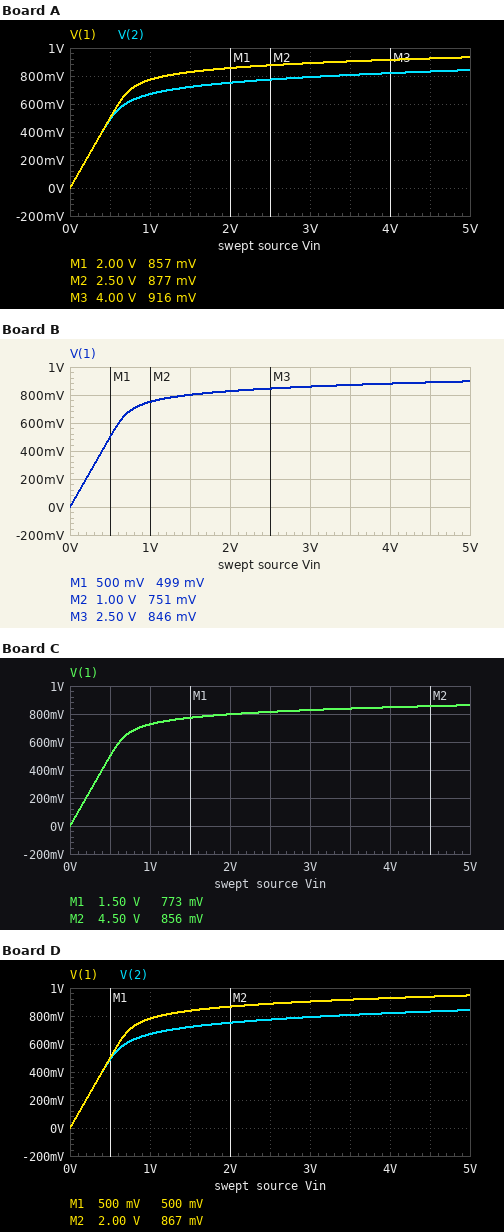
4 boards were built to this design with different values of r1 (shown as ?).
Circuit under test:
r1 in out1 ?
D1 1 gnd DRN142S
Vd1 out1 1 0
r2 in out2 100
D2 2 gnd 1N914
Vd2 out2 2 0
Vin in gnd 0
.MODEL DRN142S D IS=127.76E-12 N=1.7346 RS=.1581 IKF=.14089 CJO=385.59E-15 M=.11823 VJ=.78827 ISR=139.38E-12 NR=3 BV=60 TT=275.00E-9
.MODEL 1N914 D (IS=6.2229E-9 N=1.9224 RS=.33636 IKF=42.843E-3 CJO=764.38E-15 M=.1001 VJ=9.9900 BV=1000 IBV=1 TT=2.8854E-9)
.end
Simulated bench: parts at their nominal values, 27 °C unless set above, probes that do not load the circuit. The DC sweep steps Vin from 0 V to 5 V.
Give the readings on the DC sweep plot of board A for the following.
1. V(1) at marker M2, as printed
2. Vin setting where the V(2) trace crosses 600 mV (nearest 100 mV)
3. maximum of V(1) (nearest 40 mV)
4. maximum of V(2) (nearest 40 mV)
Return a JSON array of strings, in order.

["877 mV", "700 mV", "920 mV", "840 mV"]
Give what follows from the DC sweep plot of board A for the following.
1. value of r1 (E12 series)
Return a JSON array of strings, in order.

["68 Ω"]
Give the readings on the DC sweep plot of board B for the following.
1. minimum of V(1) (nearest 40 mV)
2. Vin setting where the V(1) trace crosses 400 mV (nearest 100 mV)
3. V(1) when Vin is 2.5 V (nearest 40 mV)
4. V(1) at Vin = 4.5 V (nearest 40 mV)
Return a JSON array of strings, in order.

["0 V", "400 mV", "840 mV", "880 mV"]
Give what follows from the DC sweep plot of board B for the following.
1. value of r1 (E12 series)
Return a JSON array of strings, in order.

["120 Ω"]
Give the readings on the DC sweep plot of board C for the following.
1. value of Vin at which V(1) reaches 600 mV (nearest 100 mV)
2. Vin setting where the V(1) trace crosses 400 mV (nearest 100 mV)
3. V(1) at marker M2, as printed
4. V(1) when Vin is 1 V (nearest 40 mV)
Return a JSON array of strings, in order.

["600 mV", "400 mV", "856 mV", "720 mV"]
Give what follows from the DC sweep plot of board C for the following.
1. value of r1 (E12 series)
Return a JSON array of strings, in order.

["220 Ω"]
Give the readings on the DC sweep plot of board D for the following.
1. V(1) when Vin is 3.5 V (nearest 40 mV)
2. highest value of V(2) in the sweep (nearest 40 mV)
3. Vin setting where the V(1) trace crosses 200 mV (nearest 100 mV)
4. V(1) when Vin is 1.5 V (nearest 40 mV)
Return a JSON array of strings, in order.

["920 mV", "840 mV", "200 mV", "840 mV"]
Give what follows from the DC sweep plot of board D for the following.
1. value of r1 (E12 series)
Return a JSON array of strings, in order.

["56 Ω"]
